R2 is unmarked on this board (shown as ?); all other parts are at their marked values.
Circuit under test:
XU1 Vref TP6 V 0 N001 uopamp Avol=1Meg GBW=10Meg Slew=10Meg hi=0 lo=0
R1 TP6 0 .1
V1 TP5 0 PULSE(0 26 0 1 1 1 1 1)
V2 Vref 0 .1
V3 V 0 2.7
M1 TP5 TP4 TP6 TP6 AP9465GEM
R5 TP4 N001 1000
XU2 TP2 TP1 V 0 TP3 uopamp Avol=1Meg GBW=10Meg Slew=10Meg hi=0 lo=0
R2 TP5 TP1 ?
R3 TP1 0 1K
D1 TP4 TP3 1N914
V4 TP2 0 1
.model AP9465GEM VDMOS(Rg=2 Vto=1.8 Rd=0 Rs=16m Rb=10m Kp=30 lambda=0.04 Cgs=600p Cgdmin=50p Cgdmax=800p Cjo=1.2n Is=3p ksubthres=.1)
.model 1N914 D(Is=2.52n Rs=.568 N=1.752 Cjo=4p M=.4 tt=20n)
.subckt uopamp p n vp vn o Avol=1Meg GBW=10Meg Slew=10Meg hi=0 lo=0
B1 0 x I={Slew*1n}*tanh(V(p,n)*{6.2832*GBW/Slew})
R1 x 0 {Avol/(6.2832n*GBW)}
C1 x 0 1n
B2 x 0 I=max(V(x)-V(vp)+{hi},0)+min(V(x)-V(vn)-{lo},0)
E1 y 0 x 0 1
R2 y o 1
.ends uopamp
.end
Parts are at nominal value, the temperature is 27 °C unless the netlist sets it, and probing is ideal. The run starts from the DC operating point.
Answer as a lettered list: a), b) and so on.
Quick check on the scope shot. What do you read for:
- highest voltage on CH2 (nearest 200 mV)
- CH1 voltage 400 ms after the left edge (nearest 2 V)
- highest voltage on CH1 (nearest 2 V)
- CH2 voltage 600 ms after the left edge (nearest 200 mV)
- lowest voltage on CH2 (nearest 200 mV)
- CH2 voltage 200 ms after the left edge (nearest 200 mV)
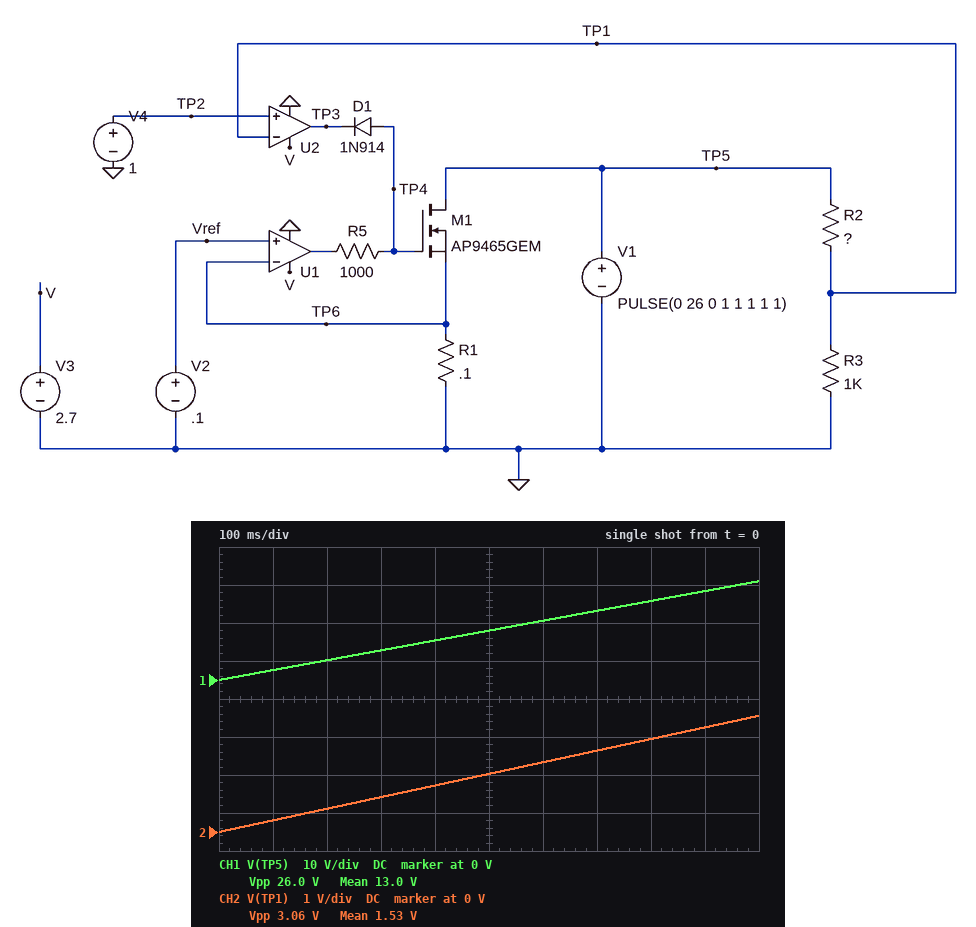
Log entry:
a) 3.0 V
b) 10 V
c) 26 V
d) 1.8 V
e) 0 V
f) 600 mV
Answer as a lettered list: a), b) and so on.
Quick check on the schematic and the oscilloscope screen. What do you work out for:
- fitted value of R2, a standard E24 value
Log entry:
a) 7.5 kΩ
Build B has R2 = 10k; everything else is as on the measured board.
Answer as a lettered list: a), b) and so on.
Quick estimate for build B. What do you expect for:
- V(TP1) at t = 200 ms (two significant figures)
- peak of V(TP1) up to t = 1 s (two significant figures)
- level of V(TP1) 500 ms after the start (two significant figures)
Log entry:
a) 470 mV
b) 2.4 V
c) 1.2 V
